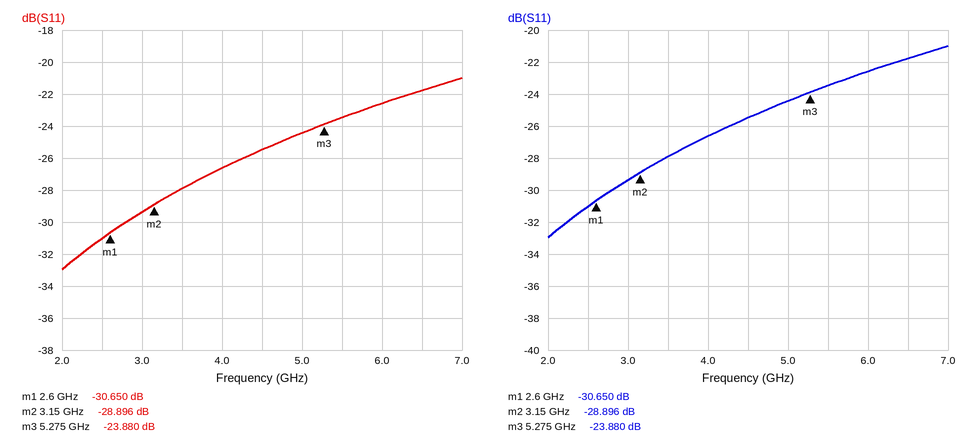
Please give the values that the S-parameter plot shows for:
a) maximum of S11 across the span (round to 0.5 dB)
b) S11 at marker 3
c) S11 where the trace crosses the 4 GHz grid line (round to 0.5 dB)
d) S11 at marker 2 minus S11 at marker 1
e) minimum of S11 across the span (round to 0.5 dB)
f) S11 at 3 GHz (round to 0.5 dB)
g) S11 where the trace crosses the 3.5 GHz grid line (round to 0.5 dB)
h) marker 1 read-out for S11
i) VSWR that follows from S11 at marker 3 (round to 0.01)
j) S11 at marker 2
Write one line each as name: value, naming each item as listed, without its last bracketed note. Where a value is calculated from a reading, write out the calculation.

maximum of S11 across the span: -21.0 dB
S11 at marker 3: -23.880 dB
S11 where the trace crosses the 4 GHz grid line: -26.5 dB
S11 at marker 2 minus S11 at marker 1: -28.896 − (-30.65) = 1.754 dB
minimum of S11 across the span: -33.0 dB
S11 at 3 GHz: -29.5 dB
S11 where the trace crosses the 3.5 GHz grid line: -28.0 dB
marker 1 read-out for S11: -30.650 dB
VSWR that follows from S11 at marker 3: (1 + 0.0640)/(1 − 0.0640) ≈ 1.14
S11 at marker 2: -28.896 dB
